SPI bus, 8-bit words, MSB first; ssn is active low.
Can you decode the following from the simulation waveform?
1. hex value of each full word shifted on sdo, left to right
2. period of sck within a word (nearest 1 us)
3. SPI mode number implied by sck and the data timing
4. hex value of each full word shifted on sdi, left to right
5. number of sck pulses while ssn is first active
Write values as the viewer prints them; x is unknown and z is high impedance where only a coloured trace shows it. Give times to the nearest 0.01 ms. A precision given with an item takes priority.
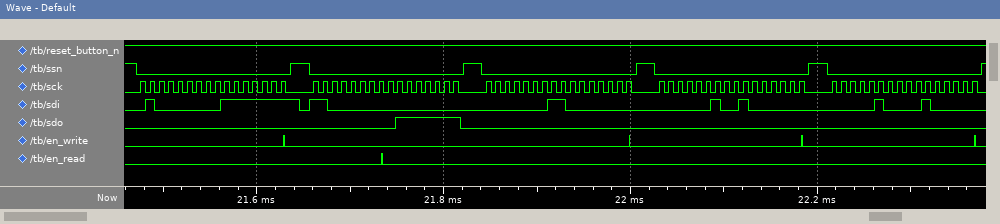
00, 00, 00, 7F, 00, 00, 00, 00, 00, 00
10 us
0
40, 7F, C0, 00, 01, 80, 02, 40, 04, 20
16
